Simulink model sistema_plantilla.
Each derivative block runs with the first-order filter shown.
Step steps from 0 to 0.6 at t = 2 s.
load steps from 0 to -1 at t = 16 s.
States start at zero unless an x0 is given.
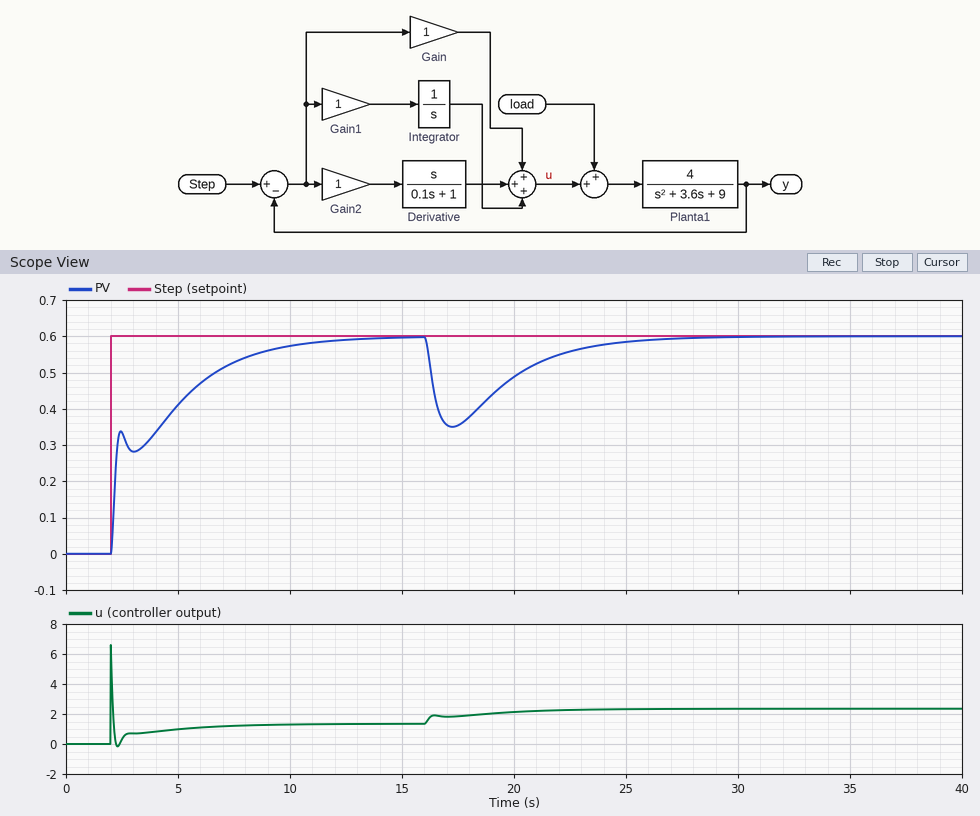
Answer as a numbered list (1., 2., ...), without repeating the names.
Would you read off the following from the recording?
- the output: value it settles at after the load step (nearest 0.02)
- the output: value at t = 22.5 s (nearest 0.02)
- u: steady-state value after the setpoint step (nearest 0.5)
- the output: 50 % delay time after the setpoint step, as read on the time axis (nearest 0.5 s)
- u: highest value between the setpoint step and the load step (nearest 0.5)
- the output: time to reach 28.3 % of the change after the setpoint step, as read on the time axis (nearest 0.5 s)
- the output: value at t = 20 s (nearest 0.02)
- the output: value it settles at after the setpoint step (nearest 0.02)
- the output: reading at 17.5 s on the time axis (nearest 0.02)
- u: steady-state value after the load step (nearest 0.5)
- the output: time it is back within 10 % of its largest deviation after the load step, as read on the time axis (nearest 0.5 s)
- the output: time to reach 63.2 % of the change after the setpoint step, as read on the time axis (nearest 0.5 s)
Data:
1. 0.60
2. 0.56
3. 1.5
4. 2.5 s
5. 6.5
6. 2.0 s
7. 0.48
8. 0.60
9. 0.36
10. 2.5
11. 24.0 s
12. 4.5 s
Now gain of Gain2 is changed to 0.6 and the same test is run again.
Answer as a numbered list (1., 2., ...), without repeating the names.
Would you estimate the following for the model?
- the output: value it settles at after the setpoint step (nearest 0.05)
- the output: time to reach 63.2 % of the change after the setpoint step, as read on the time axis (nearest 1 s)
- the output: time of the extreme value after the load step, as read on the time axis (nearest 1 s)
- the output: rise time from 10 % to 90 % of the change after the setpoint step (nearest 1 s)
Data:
1. 0.60
2. 4 s
3. 17 s
4. 6 s
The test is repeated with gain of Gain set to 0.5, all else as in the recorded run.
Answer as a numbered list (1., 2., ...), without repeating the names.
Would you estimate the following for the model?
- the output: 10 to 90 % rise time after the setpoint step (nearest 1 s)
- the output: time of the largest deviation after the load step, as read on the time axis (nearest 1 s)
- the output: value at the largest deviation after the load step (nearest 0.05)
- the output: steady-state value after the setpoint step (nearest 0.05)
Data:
1. 5 s
2. 17 s
3. 0.30
4. 0.60
